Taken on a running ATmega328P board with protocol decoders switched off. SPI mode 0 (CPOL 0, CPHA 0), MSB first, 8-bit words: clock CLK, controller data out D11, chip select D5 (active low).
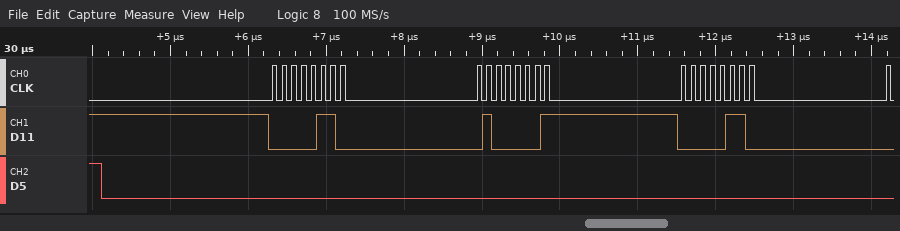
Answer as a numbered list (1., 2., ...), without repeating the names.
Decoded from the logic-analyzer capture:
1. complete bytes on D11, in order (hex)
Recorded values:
1. 0x06 0x41 0x06
